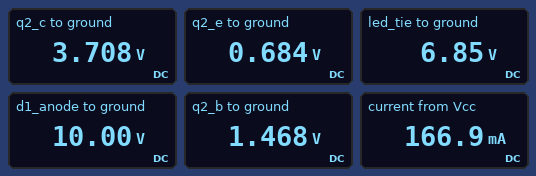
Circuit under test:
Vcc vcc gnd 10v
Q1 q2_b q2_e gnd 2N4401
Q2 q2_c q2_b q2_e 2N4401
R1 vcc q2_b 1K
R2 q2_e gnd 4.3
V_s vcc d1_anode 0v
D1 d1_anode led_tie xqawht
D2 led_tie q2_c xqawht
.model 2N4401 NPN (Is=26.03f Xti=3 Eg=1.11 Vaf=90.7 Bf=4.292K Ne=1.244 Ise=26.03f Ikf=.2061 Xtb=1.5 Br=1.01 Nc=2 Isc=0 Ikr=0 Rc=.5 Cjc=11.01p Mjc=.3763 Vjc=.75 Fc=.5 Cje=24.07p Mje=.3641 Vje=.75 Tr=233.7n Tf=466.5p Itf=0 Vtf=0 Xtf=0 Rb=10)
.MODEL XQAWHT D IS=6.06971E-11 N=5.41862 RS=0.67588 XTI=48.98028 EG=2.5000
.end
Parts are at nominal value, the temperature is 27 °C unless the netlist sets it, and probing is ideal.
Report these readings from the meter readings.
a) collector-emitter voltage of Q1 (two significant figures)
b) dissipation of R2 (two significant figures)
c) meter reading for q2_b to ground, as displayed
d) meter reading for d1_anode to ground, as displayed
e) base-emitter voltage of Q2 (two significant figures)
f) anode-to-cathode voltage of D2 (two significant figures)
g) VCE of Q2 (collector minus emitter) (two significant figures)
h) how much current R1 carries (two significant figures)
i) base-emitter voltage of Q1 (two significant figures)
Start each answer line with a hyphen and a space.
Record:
- 1.5 V
- 110 mW
- 1.468 V
- 10.00 V
- 780 mV
- 3.1 V
- 3.0 V
- 8.5 mA
- 680 mV
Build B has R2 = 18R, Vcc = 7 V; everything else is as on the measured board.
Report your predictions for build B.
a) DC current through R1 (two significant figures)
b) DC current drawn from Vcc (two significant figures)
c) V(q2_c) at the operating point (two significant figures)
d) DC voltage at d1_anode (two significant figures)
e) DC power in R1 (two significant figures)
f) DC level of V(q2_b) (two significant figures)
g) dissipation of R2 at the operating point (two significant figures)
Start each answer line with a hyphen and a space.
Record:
- 5.6 mA
- 43 mA
- 1.3 V
- 7.0 V
- 31 mW
- 1.4 V
- 25 mW
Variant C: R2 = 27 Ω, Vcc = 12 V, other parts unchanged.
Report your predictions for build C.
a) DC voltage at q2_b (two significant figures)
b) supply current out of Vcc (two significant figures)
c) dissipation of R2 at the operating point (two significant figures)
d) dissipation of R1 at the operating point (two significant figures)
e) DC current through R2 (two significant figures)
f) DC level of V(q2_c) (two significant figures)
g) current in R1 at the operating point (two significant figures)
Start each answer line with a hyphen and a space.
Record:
- 1.4 V
- 36 mA
- 18 mW
- 110 mW
- 26 mA
- 6.4 V
- 11 mA
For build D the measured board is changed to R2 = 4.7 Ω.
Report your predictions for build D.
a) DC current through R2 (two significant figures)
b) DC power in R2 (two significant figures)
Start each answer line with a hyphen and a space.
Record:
- 150 mA
- 100 mW
